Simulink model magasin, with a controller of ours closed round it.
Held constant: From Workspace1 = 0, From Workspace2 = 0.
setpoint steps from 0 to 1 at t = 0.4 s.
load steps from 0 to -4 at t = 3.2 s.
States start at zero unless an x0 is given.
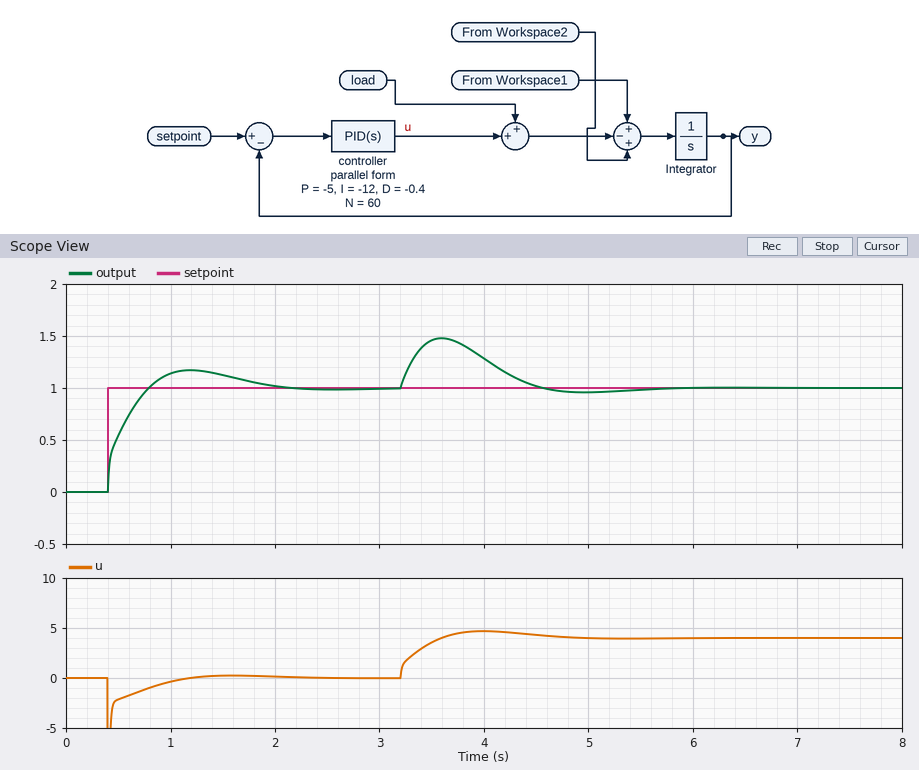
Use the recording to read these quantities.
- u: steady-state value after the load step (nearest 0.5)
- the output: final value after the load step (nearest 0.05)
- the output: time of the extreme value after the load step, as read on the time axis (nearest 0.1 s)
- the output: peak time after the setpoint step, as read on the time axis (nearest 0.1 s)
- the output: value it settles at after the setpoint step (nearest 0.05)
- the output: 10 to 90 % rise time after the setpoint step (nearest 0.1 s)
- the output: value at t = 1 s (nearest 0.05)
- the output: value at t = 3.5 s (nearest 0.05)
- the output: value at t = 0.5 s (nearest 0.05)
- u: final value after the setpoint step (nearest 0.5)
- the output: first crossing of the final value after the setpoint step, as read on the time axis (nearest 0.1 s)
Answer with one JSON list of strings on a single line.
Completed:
["4.0", "1.00", "3.6 s", "1.2 s", "1.00", "0.3 s", "1.15", "1.45", "0.55", "0.0", "0.8 s"]
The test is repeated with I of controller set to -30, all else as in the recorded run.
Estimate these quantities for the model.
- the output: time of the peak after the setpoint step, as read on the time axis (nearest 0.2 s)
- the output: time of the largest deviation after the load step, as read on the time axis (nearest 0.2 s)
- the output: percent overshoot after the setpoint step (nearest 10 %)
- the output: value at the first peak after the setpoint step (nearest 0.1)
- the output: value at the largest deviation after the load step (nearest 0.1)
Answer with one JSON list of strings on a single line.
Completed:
["1.0 s", "3.4 s", "30 %", "1.3", "1.4"]
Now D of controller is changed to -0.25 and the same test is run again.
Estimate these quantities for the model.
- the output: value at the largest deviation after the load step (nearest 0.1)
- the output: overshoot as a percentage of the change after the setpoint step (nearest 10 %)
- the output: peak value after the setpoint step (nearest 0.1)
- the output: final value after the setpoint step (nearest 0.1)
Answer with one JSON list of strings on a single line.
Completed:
["1.5", "20 %", "1.2", "1.0"]
